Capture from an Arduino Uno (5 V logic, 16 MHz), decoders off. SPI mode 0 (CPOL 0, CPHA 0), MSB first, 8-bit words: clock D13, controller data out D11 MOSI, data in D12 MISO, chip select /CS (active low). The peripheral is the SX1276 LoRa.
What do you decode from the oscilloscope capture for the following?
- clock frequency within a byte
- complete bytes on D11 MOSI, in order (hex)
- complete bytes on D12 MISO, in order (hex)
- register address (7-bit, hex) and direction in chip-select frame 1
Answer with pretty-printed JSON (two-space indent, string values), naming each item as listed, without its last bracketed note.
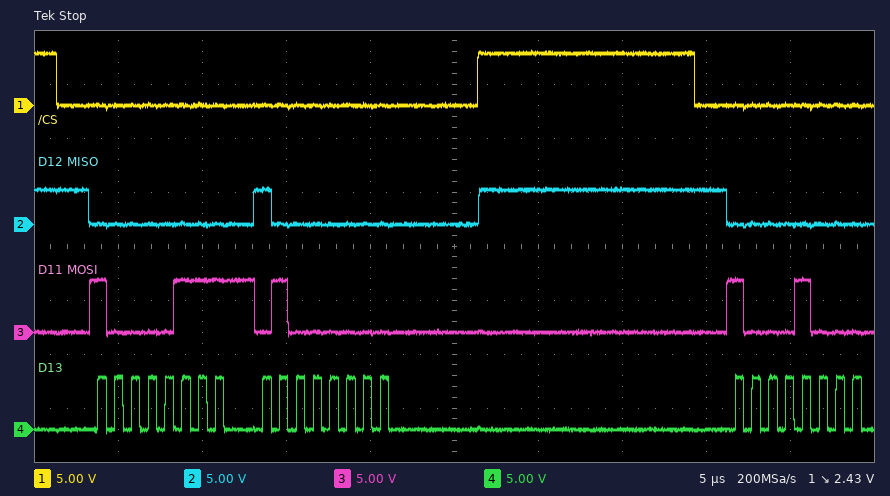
{
  "clock frequency within a byte": "1 MHz",
  "complete bytes on D11 MOSI, in order": "87 40 88",
  "complete bytes on D12 MISO, in order": "00 80 00",
  "register address (7-bit, hex) and direction in chip-select frame 1": "0x07 write"
}
